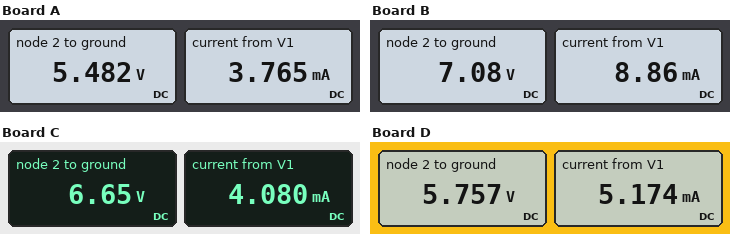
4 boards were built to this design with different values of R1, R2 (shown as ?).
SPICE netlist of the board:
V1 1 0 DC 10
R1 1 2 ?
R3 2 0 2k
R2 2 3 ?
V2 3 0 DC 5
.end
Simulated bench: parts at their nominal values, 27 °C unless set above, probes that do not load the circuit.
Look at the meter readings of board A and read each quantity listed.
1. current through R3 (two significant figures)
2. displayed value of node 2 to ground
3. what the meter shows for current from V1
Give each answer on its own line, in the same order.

2.7 mA
5.482 V
3.765 mA
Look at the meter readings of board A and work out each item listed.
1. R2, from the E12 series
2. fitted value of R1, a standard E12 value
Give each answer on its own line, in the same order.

470 Ω
1.2 kΩ
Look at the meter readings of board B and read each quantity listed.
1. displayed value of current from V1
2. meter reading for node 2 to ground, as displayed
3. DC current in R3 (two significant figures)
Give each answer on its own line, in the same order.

8.86 mA
7.08 V
3.5 mA
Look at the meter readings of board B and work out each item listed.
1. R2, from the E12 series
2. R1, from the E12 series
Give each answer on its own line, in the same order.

390 Ω
330 Ω
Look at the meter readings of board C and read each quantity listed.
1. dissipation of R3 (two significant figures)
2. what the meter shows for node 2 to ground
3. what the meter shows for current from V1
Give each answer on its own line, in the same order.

22 mW
6.65 V
4.080 mA
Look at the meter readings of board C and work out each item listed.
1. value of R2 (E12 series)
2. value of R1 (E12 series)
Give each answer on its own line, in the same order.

2.2 kΩ
820 Ω
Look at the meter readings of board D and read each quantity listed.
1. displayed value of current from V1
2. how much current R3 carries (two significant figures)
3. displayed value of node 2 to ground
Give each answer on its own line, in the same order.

5.174 mA
2.9 mA
5.757 V
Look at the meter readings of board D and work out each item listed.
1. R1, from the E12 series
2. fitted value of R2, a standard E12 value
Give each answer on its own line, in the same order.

820 Ω
330 Ω
